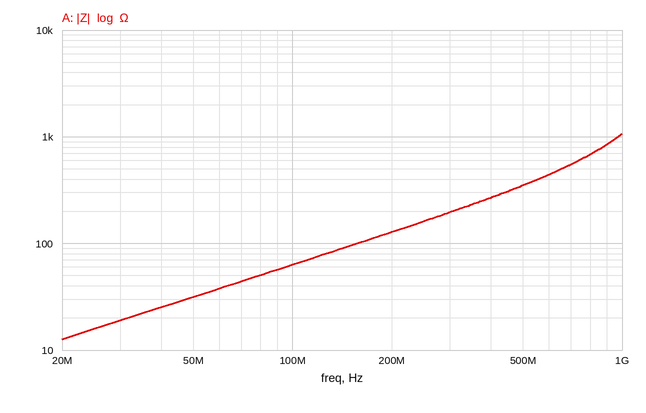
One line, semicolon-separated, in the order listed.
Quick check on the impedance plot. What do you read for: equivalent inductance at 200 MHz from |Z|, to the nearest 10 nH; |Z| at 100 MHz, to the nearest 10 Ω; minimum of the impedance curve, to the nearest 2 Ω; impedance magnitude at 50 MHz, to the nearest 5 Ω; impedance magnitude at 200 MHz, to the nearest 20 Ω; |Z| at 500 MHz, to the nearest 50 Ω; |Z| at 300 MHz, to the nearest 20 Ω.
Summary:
100 nH; 60 Ω; 12 Ω; 30 Ω; 120 Ω; 350 Ω; 200 Ω
